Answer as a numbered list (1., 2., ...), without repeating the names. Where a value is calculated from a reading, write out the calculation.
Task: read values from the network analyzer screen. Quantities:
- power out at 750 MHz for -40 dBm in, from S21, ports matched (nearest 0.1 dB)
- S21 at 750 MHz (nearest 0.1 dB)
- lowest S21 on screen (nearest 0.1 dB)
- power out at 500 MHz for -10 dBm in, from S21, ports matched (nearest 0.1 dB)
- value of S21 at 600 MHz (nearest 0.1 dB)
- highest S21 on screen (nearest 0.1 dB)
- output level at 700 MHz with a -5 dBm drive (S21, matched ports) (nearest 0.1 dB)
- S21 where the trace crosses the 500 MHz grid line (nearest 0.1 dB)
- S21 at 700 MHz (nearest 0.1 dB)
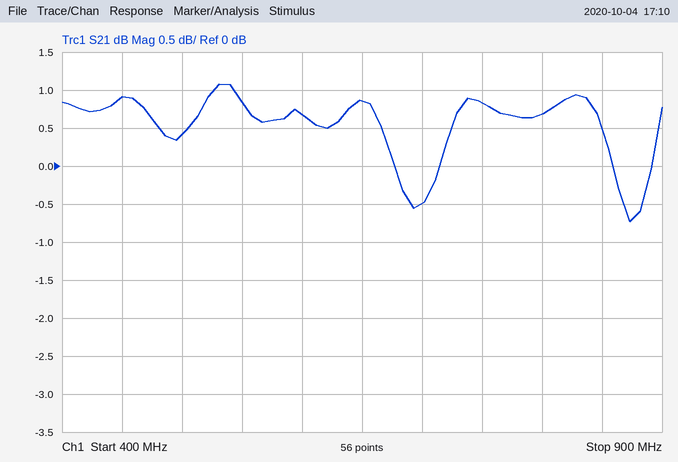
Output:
1. -40 dBm + (0.8 dB) = -39.2 dBm
2. 0.8 dB
3. -0.7 dB
4. -10 dBm + (0.4 dB) = -9.6 dBm
5. 0.7 dB
6. 1.1 dB
7. -5 dBm + (-0.5 dB) = -5.5 dBm
8. 0.4 dB
9. -0.5 dB
